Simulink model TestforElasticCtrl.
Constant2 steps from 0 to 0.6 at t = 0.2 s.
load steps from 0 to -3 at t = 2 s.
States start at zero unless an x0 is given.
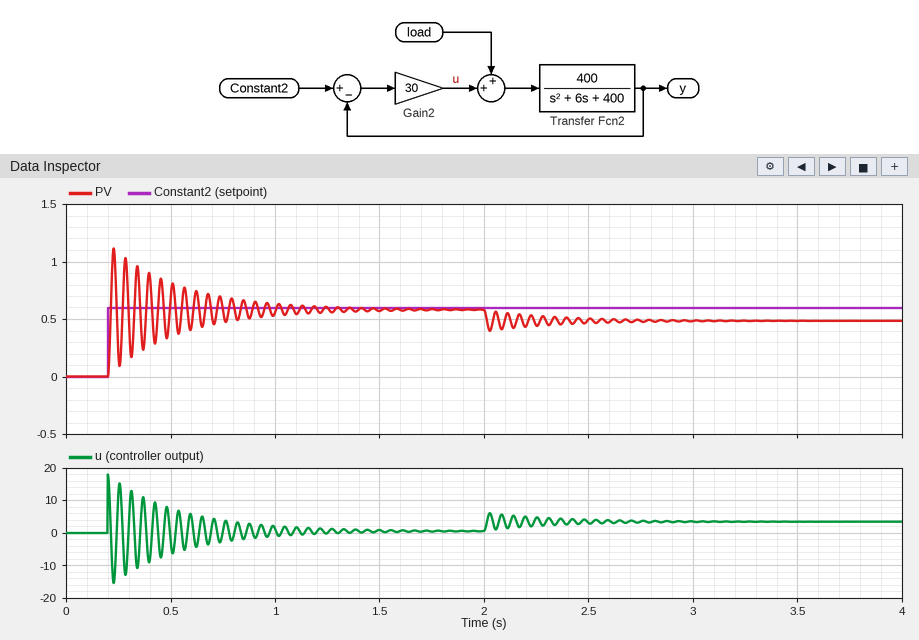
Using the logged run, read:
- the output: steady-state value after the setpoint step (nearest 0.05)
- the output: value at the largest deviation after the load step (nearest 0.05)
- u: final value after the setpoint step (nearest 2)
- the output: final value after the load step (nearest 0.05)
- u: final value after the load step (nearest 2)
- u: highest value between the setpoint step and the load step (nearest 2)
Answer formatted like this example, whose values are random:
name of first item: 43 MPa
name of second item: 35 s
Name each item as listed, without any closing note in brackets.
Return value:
the output: steady-state value after the setpoint step: 0.60
the output: value at the largest deviation after the load step: 0.40
u: final value after the setpoint step: 0
the output: final value after the load step: 0.50
u: final value after the load step: 4
u: highest value between the setpoint step and the load step: 18
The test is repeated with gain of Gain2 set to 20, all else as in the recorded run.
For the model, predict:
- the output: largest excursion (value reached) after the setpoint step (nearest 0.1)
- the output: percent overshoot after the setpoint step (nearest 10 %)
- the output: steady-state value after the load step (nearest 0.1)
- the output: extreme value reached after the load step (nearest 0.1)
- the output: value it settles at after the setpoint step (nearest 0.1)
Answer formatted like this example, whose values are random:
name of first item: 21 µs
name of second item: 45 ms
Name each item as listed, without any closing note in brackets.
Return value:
the output: largest excursion (value reached) after the setpoint step: 1.1
the output: percent overshoot after the setpoint step: 90 %
the output: steady-state value after the load step: 0.4
the output: extreme value reached after the load step: 0.3
the output: value it settles at after the setpoint step: 0.6
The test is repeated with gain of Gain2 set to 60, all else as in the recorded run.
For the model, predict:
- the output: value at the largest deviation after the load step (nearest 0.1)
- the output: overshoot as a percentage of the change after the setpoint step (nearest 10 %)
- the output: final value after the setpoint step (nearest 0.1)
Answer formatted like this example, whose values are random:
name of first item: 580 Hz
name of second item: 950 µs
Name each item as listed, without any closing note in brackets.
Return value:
the output: value at the largest deviation after the load step: 0.5
the output: overshoot as a percentage of the change after the setpoint step: 90 %
the output: final value after the setpoint step: 0.6
